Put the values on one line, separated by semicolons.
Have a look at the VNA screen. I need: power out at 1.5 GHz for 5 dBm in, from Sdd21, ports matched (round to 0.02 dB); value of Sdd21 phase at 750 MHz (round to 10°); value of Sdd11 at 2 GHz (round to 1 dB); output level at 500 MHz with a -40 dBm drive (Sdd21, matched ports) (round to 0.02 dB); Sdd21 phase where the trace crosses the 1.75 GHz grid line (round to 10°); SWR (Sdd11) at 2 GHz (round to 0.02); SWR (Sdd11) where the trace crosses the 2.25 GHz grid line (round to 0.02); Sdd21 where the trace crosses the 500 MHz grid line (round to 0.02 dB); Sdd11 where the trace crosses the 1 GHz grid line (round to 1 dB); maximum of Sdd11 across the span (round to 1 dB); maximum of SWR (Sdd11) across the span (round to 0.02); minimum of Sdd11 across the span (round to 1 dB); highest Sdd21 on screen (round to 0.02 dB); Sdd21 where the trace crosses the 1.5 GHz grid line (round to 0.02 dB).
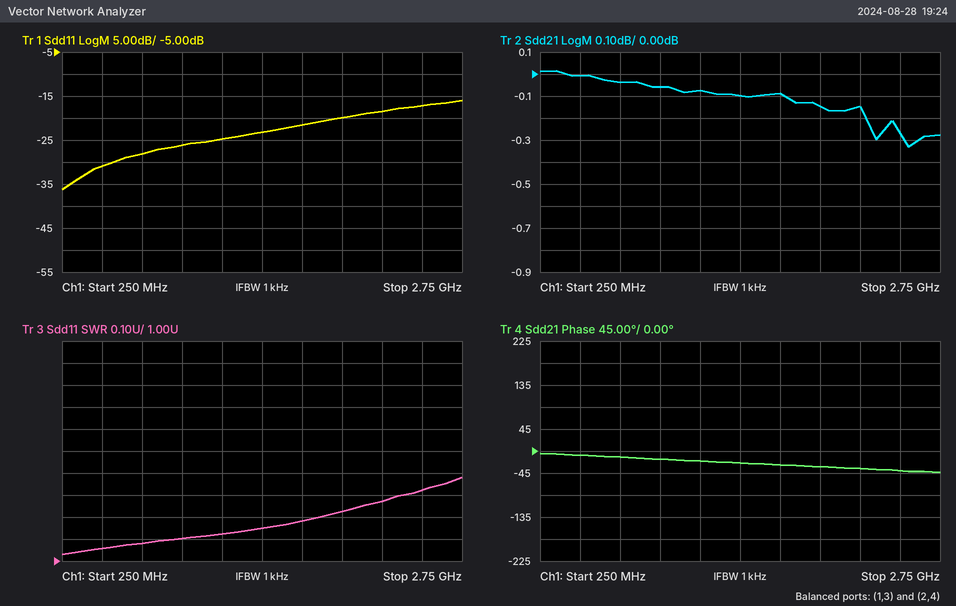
4.90 dBm; -10°; -20 dB; -40.00 dBm; -30°; 1.22; 1.28; 0.00 dB; -26 dB; -16 dB; 1.38; -36 dB; 0.02 dB; -0.10 dB
